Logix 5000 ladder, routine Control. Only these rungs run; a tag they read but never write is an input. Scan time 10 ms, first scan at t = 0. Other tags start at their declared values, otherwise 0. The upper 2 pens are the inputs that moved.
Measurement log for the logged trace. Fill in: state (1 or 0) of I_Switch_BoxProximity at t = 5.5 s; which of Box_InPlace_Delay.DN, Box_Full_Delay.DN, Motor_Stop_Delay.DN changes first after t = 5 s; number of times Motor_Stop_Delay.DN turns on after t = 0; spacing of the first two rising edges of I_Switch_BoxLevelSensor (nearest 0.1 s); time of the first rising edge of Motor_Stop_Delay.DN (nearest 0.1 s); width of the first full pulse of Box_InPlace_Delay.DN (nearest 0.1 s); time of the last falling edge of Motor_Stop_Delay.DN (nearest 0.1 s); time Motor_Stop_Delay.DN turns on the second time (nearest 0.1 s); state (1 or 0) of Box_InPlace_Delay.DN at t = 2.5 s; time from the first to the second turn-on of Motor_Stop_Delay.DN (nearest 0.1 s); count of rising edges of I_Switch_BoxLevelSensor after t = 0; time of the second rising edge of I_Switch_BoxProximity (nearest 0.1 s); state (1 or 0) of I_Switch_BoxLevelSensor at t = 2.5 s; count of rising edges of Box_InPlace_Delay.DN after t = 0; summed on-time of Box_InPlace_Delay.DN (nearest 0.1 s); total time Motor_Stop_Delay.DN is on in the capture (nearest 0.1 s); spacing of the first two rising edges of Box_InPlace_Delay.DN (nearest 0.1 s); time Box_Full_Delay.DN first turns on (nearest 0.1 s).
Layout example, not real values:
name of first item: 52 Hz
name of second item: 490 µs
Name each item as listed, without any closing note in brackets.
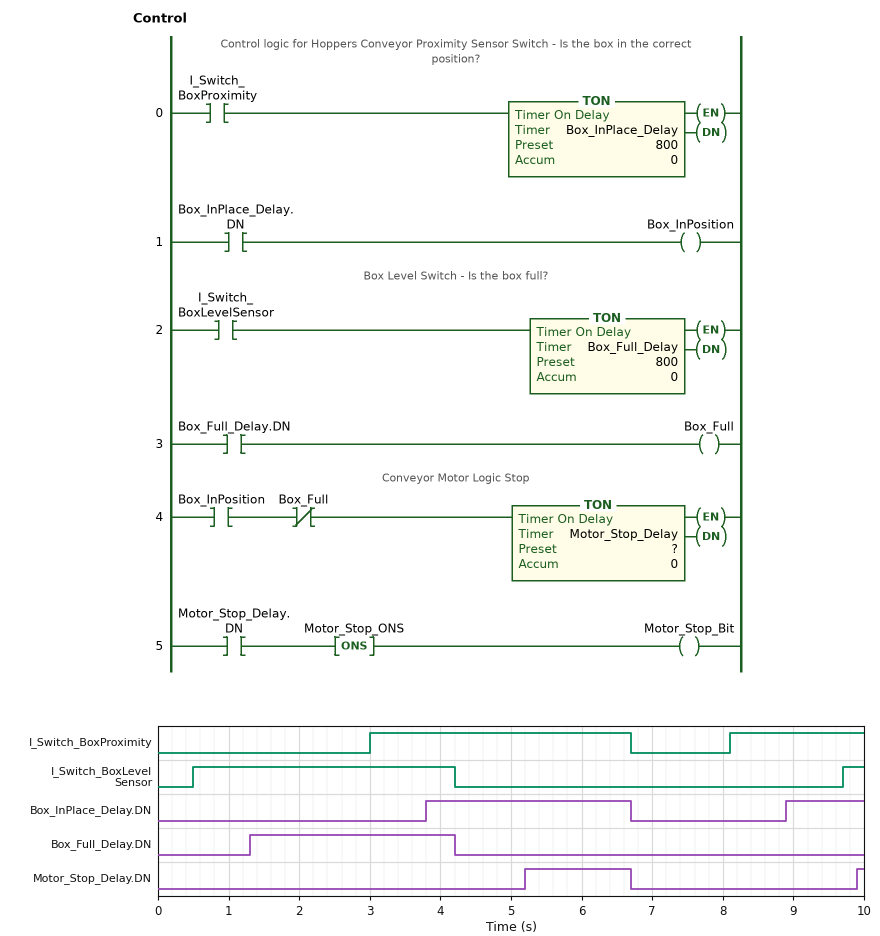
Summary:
state (1 or 0) of I_Switch_BoxProximity at t = 5.5 s: 1
which of Box_InPlace_Delay.DN, Box_Full_Delay.DN, Motor_Stop_Delay.DN changes first after t = 5 s: Motor_Stop_Delay.DN
number of times Motor_Stop_Delay.DN turns on after t = 0: 2
spacing of the first two rising edges of I_Switch_BoxLevelSensor: 9.2 s
time of the first rising edge of Motor_Stop_Delay.DN: 5.2 s
width of the first full pulse of Box_InPlace_Delay.DN: 2.9 s
time of the last falling edge of Motor_Stop_Delay.DN: 6.7 s
time Motor_Stop_Delay.DN turns on the second time: 9.9 s
state (1 or 0) of Box_InPlace_Delay.DN at t = 2.5 s: 0
time from the first to the second turn-on of Motor_Stop_Delay.DN: 4.7 s
count of rising edges of I_Switch_BoxLevelSensor after t = 0: 2
time of the second rising edge of I_Switch_BoxProximity: 8.1 s
state (1 or 0) of I_Switch_BoxLevelSensor at t = 2.5 s: 1
count of rising edges of Box_InPlace_Delay.DN after t = 0: 2
summed on-time of Box_InPlace_Delay.DN: 4.0 s
total time Motor_Stop_Delay.DN is on in the capture: 1.6 s
spacing of the first two rising edges of Box_InPlace_Delay.DN: 5.1 s
time Box_Full_Delay.DN first turns on: 1.3 s
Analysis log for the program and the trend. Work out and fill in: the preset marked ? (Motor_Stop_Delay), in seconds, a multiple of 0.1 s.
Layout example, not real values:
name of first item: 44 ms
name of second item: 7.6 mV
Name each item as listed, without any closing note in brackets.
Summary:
the preset marked ? (Motor_Stop_Delay), in seconds, a multiple of 0.1 s: 1.0 s
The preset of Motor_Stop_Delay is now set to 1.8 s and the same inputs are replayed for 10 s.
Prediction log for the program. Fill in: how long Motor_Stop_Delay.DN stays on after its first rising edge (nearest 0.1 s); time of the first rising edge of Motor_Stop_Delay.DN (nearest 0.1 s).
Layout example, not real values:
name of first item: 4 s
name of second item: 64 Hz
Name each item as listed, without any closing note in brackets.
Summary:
how long Motor_Stop_Delay.DN stays on after its first rising edge: 0.7 s
time of the first rising edge of Motor_Stop_Delay.DN: 6.0 s
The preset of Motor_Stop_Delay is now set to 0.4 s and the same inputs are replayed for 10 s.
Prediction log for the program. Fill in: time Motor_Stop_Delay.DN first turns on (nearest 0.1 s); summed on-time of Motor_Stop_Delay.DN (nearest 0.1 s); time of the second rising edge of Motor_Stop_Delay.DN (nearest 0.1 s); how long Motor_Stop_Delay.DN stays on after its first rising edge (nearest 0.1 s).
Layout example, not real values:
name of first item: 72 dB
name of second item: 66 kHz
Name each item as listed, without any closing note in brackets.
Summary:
time Motor_Stop_Delay.DN first turns on: 4.6 s
summed on-time of Motor_Stop_Delay.DN: 2.8 s
time of the second rising edge of Motor_Stop_Delay.DN: 9.3 s
how long Motor_Stop_Delay.DN stays on after its first rising edge: 2.1 s
